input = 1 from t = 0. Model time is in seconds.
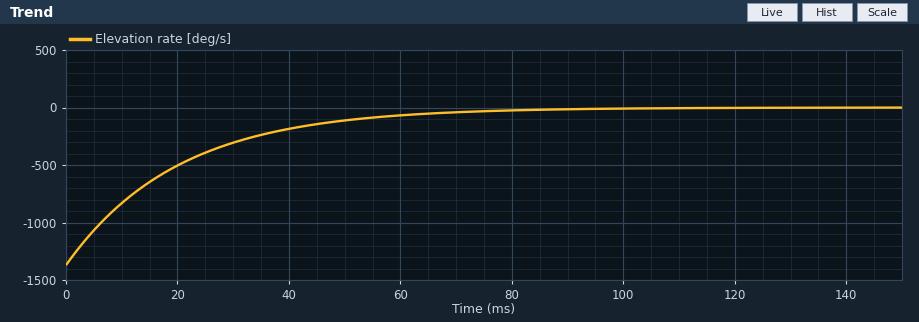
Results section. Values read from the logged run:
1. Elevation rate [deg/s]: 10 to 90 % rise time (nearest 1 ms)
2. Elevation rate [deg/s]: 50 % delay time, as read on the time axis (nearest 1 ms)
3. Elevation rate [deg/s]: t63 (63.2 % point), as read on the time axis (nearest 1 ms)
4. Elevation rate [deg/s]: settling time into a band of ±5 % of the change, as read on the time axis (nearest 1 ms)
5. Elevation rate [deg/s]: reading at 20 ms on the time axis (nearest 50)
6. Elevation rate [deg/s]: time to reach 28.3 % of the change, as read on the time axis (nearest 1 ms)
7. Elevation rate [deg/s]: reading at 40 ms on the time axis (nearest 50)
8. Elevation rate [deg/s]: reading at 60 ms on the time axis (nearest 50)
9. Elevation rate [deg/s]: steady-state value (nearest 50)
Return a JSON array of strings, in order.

["44 ms", "14 ms", "20 ms", "60 ms", "-500", "7 ms", "-200", "-50", "0"]
